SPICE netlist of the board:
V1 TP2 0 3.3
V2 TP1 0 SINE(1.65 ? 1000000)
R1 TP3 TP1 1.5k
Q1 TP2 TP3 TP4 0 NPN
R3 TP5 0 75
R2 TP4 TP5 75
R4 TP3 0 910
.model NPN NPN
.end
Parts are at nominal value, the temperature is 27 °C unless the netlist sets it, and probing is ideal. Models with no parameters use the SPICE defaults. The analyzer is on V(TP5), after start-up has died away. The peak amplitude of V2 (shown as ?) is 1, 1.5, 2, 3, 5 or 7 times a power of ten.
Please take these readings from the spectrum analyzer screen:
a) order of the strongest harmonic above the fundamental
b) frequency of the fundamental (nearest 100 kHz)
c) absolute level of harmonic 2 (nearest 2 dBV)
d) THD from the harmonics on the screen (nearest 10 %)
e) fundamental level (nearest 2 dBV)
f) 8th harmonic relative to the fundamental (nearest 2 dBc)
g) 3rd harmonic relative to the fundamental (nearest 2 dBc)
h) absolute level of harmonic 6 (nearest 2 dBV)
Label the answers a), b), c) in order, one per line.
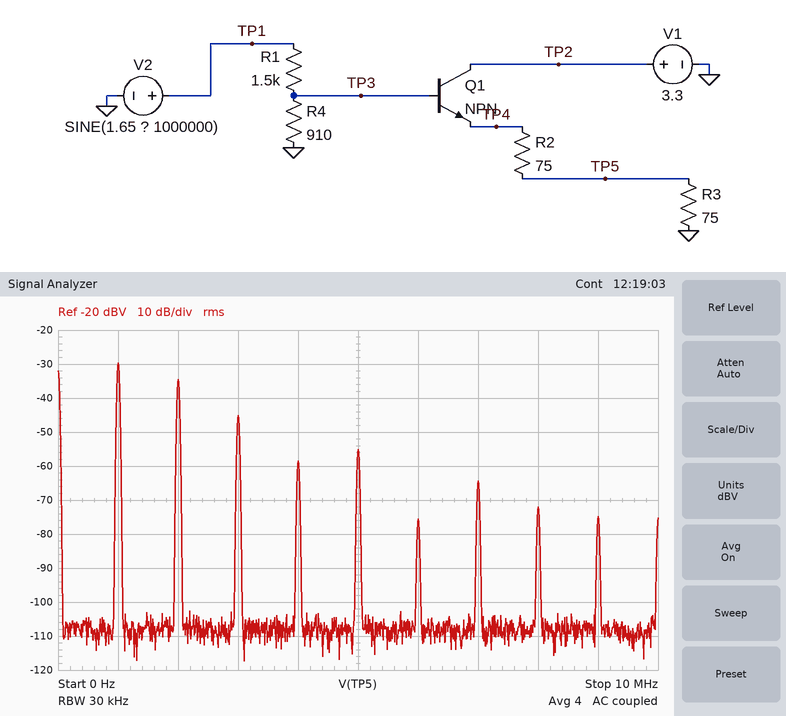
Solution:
a) 2
b) 1.0 MHz
c) -34 dBV
d) 60 %
e) -30 dBV
f) -42 dBc
g) -16 dBc
h) -76 dBV
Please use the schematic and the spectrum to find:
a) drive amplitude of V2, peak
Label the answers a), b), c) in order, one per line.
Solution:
a) 1 V
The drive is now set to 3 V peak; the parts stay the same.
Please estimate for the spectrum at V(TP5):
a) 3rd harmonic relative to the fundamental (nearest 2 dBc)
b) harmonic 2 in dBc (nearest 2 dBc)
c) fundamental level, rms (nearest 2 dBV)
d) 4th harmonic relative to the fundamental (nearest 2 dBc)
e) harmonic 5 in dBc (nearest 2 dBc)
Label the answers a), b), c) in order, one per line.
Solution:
a) -24 dBc
b) -6 dBc
c) -16 dBV
d) -22 dBc
e) -30 dBc
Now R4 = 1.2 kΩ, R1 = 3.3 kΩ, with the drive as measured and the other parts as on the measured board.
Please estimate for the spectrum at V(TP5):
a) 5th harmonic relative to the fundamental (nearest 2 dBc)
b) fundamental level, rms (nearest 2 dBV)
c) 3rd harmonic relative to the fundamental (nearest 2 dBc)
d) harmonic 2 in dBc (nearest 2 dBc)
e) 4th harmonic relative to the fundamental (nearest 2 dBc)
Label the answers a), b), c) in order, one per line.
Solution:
a) -12 dBc
b) -62 dBV
c) -4 dBc
d) -2 dBc
e) -8 dBc
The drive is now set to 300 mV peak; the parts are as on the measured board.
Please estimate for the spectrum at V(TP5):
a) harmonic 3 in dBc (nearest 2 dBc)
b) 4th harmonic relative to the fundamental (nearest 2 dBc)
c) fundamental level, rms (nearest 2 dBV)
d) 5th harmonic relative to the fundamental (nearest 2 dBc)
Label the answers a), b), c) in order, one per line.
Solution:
a) -12 dBc
b) -24 dBc
c) -52 dBV
d) -52 dBc
